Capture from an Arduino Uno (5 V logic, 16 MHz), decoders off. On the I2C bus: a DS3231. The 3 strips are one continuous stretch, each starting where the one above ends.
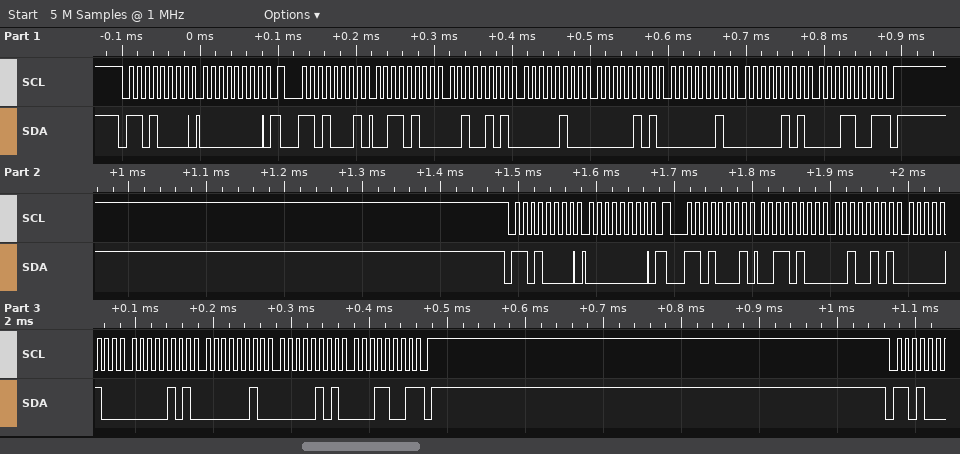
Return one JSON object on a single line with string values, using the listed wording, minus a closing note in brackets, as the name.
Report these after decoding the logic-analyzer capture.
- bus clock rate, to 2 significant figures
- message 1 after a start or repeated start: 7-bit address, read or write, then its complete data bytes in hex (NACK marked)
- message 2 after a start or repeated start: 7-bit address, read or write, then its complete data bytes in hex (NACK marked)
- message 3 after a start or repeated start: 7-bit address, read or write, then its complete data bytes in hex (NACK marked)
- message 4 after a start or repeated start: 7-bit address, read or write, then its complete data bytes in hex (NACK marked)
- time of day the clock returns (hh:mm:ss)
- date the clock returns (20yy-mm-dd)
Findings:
{"bus clock rate, to 2 significant figures": "100 kHz", "message 1 after a start or repeated start: 7-bit address, read or write, then its complete data bytes in hex": "0x68 write: 00", "message 2 after a start or repeated start: 7-bit address, read or write, then its complete data bytes in hex": "0x68 read: 34 25 04 05 02 05 19 NACK", "message 3 after a start or repeated start: 7-bit address, read or write, then its complete data bytes in hex": "0x68 write: 00", "message 4 after a start or repeated start: 7-bit address, read or write, then its complete data bytes in hex": "0x68 read: 34 25 04 05 02 05 19 NACK", "time of day the clock returns": "04:25:34", "date the clock returns": "2019-05-02"}
